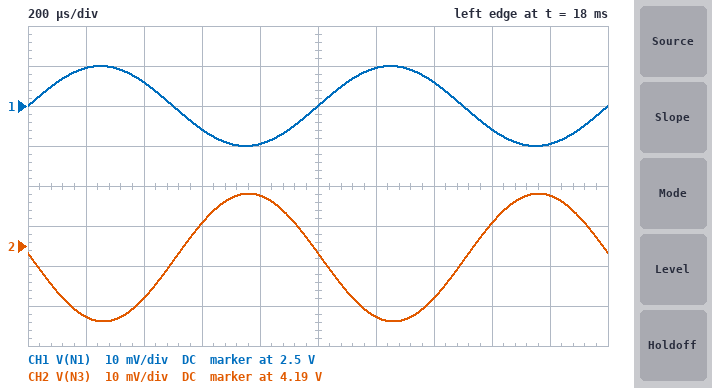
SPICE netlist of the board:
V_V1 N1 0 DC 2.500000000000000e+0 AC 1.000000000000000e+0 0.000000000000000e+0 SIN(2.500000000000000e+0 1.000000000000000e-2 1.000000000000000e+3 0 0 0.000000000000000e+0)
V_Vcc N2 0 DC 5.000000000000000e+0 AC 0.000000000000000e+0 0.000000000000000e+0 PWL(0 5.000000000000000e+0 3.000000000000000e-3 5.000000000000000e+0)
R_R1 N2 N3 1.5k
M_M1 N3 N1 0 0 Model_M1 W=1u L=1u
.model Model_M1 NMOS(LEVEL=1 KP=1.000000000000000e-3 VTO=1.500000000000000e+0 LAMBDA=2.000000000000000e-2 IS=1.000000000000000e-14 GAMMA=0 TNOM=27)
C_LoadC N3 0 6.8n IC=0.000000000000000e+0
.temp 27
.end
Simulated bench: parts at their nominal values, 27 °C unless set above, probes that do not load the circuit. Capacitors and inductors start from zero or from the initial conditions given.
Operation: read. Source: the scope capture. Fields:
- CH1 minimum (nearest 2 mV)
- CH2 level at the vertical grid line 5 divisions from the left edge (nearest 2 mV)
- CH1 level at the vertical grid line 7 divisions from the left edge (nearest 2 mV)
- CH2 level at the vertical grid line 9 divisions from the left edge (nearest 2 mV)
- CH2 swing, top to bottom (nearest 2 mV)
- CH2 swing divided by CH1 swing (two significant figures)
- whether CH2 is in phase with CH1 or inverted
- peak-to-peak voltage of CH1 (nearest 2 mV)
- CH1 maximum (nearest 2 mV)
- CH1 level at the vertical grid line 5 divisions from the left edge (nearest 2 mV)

2.490 V
4.188 V
2.506 V
4.202 V
32 mV
1.6
inverted
20 mV
2.510 V
2.500 V
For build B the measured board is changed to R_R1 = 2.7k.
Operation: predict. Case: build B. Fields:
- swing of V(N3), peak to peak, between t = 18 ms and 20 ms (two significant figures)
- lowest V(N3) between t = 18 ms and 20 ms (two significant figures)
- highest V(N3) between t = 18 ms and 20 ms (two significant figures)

56 mV
3.5 V
3.6 V
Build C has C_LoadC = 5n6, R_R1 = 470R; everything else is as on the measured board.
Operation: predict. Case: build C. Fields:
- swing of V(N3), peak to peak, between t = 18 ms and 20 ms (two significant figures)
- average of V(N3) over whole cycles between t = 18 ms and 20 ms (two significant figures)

10 mV
4.7 V
